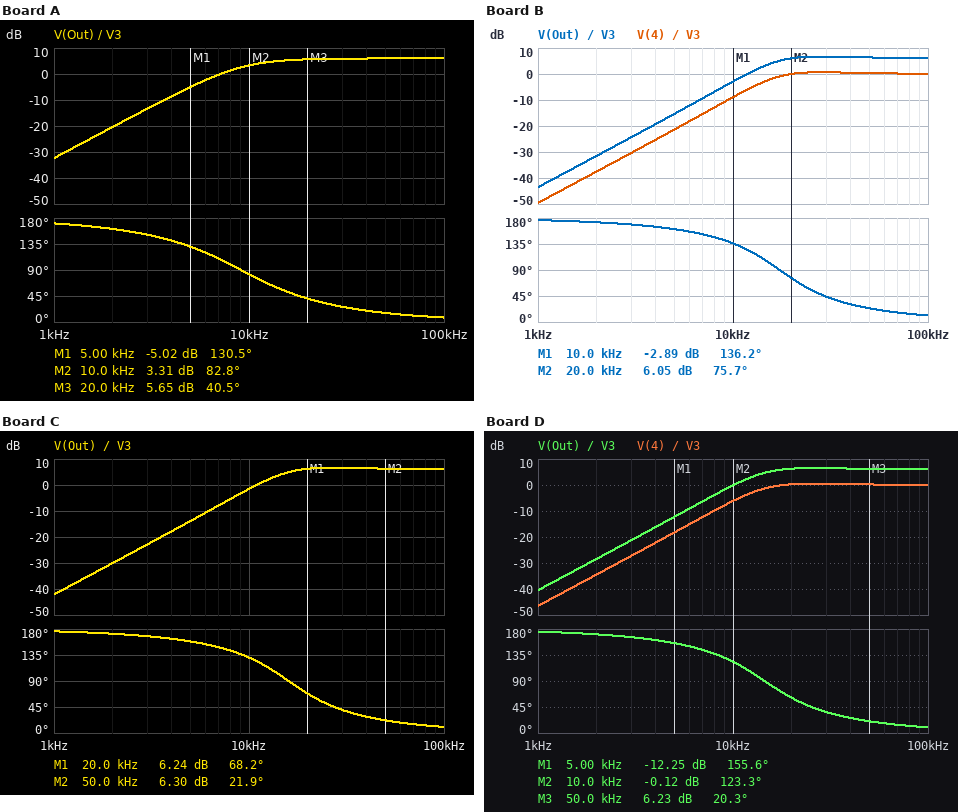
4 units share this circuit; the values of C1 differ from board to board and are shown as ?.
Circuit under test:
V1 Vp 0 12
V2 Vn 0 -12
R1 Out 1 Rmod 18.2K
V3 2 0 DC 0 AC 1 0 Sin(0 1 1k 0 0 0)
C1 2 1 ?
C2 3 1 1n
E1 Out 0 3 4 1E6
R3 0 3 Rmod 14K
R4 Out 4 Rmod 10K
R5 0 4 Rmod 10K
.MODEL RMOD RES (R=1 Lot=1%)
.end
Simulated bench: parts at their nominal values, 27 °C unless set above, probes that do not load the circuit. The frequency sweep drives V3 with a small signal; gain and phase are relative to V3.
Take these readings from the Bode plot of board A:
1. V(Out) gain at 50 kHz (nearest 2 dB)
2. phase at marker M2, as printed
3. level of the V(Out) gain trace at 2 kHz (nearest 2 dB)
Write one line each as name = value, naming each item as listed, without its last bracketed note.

V(Out) gain at 50 kHz = 6 dB
phase at marker M2, as printed = 82.8 deg
level of the V(Out) gain trace at 2 kHz = -20 dB
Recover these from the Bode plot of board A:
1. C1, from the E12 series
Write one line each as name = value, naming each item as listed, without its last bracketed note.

C1, from the E12 series = 1.2 nF
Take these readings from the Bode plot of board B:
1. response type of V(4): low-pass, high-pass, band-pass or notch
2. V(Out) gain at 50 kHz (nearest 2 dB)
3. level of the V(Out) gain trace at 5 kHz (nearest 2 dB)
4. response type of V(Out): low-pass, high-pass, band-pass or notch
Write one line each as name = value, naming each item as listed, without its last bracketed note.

response type of V(4): low-pass, high-pass, band-pass or notch = high-pass
V(Out) gain at 50 kHz = 6 dB
level of the V(Out) gain trace at 5 kHz = -16 dB
response type of V(Out): low-pass, high-pass, band-pass or notch = high-pass
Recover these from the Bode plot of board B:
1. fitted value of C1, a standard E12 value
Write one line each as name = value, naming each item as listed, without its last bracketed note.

fitted value of C1, a standard E12 value = 330 pF
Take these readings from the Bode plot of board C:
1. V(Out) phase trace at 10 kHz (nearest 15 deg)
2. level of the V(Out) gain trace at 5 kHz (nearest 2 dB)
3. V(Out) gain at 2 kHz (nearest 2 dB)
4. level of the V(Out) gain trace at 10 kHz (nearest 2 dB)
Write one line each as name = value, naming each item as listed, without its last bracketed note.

V(Out) phase trace at 10 kHz = 135 deg
level of the V(Out) gain trace at 5 kHz = -14 dB
V(Out) gain at 2 kHz = -30 dB
level of the V(Out) gain trace at 10 kHz = -2 dB
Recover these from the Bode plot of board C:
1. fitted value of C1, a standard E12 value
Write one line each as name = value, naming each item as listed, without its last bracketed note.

fitted value of C1, a standard E12 value = 390 pF
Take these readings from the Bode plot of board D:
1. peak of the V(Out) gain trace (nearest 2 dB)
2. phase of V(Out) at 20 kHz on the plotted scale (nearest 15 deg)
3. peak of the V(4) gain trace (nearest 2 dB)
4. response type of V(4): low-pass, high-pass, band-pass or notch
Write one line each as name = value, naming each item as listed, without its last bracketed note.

peak of the V(Out) gain trace = 6 dB
phase of V(Out) at 20 kHz on the plotted scale = 60 deg
peak of the V(4) gain trace = 0 dB
response type of V(4): low-pass, high-pass, band-pass or notch = high-pass
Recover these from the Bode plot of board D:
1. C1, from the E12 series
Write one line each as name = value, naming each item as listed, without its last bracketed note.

C1, from the E12 series = 470 pF
